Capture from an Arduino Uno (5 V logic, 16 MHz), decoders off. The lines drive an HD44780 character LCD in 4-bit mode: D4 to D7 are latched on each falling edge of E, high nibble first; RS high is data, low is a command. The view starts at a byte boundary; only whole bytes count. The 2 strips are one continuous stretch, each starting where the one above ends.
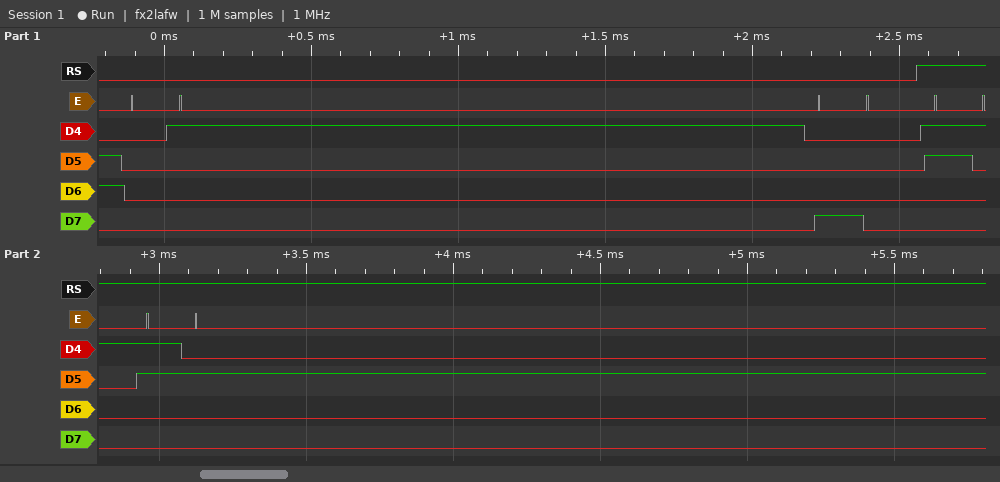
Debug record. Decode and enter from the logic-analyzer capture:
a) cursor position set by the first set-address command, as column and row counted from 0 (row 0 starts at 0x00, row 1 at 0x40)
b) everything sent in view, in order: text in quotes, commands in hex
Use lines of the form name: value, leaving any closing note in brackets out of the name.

cursor position set by the first set-address command, as column and row counted from 0: column 0, row 0
everything sent in view, in order: text in quotes, commands in hex: 0x01 0x80 "12"
